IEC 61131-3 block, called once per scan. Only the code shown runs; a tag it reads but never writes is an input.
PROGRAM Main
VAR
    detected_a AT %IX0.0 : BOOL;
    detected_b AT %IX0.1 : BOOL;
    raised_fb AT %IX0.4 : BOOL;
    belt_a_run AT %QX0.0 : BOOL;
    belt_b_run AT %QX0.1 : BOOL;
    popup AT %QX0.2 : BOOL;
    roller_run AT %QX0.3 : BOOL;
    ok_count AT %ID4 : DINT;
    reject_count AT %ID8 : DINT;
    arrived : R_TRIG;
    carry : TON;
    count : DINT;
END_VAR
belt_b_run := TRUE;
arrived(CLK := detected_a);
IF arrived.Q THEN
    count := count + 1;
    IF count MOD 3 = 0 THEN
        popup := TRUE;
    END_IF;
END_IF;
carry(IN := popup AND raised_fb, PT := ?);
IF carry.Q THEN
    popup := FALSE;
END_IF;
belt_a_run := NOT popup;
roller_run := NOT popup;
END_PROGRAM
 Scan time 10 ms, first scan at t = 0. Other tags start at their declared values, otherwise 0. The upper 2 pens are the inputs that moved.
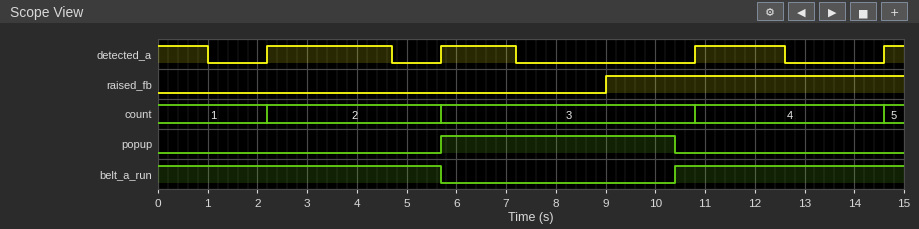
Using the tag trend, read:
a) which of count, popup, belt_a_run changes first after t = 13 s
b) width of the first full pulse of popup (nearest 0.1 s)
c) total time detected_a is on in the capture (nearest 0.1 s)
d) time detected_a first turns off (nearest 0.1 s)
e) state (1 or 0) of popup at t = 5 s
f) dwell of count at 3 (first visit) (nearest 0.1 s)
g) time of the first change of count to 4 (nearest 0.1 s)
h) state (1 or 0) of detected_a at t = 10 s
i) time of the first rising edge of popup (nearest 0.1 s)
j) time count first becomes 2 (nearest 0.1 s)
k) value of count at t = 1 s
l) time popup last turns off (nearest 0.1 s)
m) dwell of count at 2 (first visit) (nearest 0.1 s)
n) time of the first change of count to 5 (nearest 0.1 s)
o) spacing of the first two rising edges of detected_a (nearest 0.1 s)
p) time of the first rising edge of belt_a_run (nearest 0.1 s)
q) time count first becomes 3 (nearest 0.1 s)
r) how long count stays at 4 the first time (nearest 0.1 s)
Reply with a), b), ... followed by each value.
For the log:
a) count
b) 4.7 s
c) 7.2 s
d) 1.0 s
e) 0
f) 5.1 s
g) 10.8 s
h) 0
i) 5.7 s
j) 2.2 s
k) 1
l) 10.4 s
m) 3.5 s
n) 14.6 s
o) 3.5 s
p) 10.4 s
q) 5.7 s
r) 3.8 s
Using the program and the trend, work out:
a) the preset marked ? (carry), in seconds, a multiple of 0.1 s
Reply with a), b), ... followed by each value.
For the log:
a) 1.4 s
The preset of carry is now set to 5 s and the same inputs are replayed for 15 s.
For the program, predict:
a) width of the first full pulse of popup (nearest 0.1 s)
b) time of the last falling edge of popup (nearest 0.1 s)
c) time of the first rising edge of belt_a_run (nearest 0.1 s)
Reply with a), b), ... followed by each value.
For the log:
a) 8.3 s
b) 14.0 s
c) 14.0 s
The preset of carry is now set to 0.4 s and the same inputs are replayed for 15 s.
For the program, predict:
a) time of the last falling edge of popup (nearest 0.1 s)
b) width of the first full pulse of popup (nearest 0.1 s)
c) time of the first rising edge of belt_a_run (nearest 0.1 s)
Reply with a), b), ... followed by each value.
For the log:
a) 9.4 s
b) 3.7 s
c) 9.4 s
